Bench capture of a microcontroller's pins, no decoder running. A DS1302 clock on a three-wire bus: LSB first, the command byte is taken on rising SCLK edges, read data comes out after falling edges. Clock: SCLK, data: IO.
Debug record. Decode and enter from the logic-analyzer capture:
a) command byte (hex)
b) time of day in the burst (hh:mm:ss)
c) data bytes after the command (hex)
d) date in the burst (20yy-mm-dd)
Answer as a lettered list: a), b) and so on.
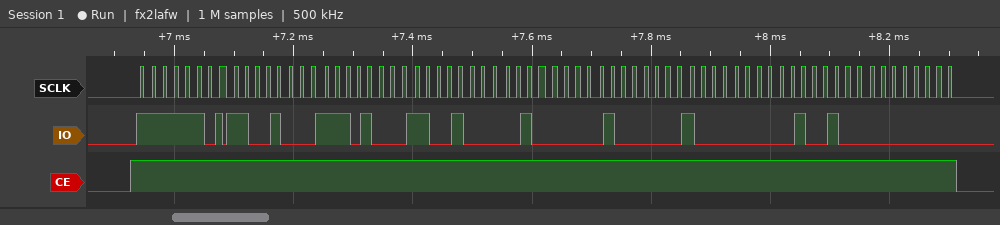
a) 0xBF
b) 13:17:13
c) 13 17 13 04 02 01 24 00
d) 2024-02-04
